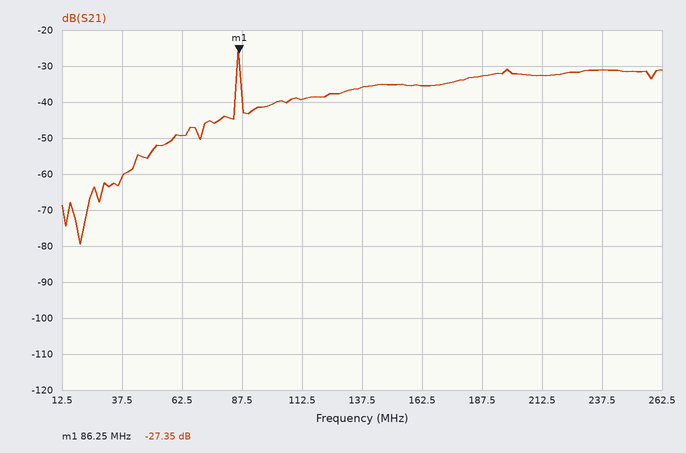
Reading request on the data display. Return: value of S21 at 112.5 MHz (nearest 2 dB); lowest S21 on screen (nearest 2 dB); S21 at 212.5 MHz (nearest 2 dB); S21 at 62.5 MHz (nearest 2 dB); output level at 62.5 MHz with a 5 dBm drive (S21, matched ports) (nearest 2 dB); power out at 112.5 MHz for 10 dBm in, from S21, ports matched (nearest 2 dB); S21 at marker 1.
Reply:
-40 dB
-80 dB
-32 dB
-50 dB
-44 dBm
-30 dBm
-27.35 dB
